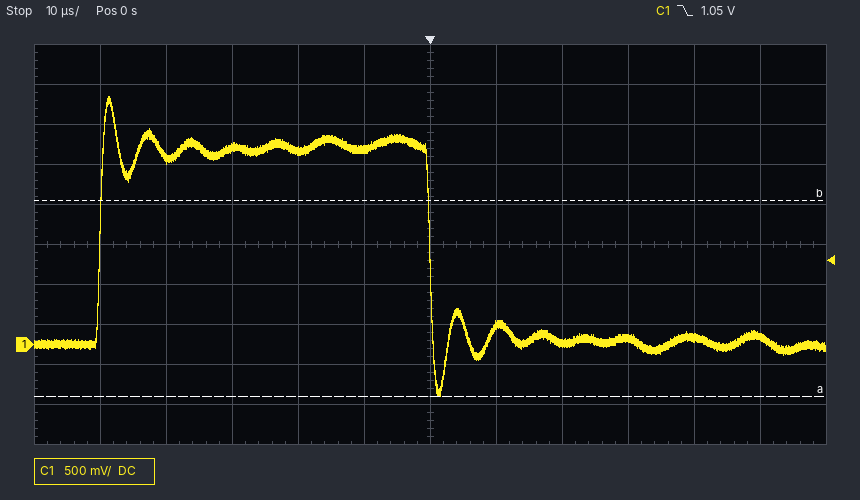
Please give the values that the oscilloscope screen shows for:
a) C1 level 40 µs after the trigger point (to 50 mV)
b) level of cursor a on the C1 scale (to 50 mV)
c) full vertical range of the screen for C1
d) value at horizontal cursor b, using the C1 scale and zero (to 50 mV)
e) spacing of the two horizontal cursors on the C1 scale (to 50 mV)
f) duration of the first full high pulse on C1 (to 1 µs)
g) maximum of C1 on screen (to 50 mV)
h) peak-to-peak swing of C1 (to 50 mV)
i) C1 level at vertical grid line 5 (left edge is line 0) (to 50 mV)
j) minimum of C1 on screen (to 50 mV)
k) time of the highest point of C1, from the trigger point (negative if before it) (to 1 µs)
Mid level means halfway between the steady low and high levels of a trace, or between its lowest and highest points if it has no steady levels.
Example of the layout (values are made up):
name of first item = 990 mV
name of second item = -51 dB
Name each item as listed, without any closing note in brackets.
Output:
C1 level 40 µs after the trigger point = 100 mV
level of cursor a on the C1 scale = -650 mV
full vertical range of the screen for C1 = 5 V
value at horizontal cursor b, using the C1 scale and zero = 1.80 V
spacing of the two horizontal cursors on the C1 scale = 2.45 V
duration of the first full high pulse on C1 = 50 µs
maximum of C1 on screen = 3.10 V
peak-to-peak swing of C1 = 3.75 V
C1 level at vertical grid line 5 (left edge is line 0) = 2.45 V
minimum of C1 on screen = -650 mV
time of the highest point of C1, from the trigger point (negative if before it) = -49 µs
